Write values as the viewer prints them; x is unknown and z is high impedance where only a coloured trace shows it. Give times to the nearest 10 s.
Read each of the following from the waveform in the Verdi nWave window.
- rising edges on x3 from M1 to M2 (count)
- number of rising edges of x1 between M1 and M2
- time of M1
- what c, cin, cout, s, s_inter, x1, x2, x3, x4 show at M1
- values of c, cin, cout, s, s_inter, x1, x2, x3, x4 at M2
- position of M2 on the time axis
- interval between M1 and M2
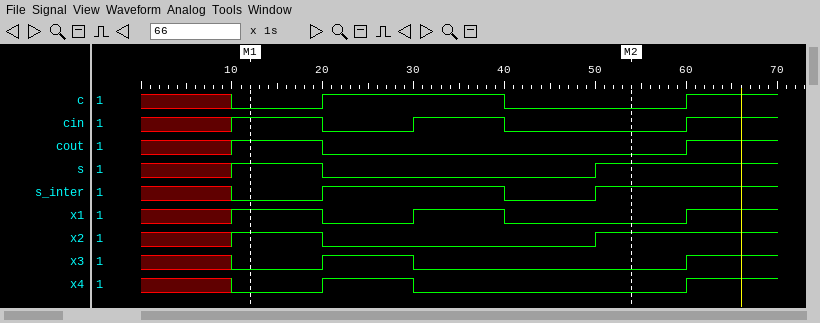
1
1
10 s
c=0, cin=1, cout=1, s=1, s_inter=0, x1=1, x2=1, x3=0, x4=0
c=0, cin=0, cout=0, s=1, s_inter=1, x1=0, x2=1, x3=0, x4=0
50 s
40 s
